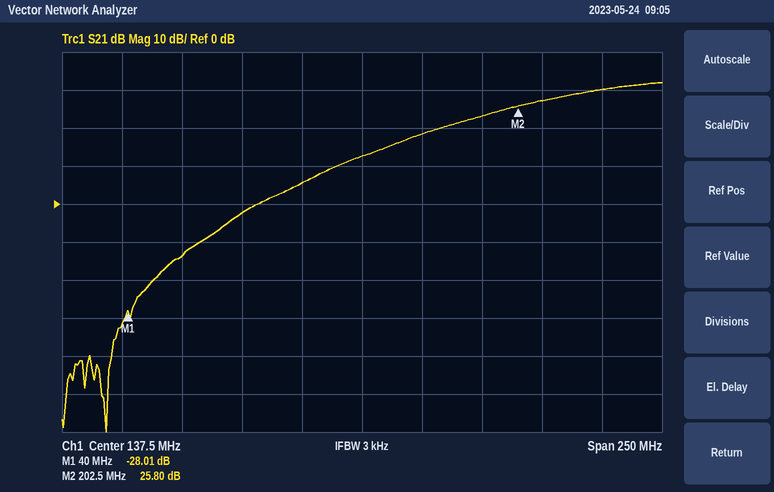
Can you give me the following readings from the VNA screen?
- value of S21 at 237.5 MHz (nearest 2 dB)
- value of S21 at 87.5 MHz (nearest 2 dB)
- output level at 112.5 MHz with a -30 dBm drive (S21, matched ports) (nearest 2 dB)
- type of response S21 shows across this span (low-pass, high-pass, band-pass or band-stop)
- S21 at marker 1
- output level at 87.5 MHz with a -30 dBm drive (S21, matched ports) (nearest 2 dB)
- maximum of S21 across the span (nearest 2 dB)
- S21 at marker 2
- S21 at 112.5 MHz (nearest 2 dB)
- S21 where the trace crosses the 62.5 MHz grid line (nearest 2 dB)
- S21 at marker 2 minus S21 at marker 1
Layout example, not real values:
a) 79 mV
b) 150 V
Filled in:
a) 30 dB
b) -2 dB
c) -24 dBm
d) high-pass
e) -28.01 dB
f) -32 dBm
g) 32 dB
h) 25.80 dB
i) 6 dB
j) -14 dB
k) 53.81 dB
